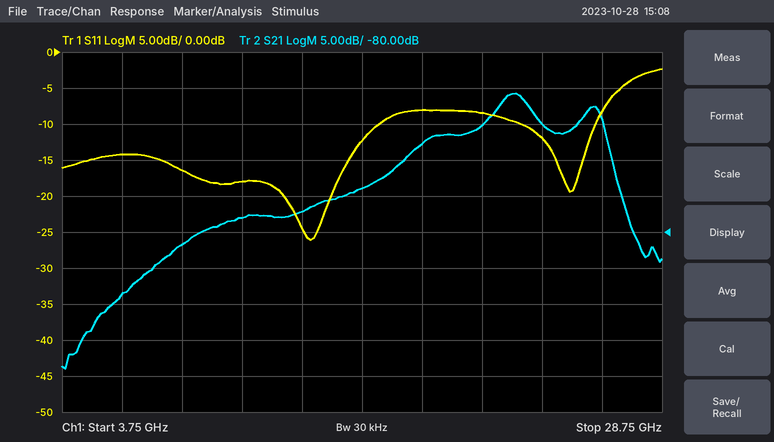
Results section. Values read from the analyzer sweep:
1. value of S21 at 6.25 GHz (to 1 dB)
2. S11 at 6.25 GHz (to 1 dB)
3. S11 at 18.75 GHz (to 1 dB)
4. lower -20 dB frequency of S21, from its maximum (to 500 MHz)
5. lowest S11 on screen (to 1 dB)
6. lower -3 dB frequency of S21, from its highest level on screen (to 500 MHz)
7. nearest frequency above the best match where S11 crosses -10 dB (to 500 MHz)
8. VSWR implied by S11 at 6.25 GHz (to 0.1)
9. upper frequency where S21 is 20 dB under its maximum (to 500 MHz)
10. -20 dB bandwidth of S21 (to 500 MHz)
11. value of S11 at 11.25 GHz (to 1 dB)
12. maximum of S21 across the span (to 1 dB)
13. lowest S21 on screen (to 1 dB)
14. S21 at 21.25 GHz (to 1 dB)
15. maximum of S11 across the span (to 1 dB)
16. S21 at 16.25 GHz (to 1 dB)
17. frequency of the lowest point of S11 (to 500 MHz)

-89 dB
-14 dB
-8 dB
9.0 GHz
-26 dB
21.5 GHz
17.0 GHz
1.5
27.5 GHz
18.5 GHz
-18 dB
-61 dB
-99 dB
-65 dB
-2 dB
-74 dB
14.0 GHz
